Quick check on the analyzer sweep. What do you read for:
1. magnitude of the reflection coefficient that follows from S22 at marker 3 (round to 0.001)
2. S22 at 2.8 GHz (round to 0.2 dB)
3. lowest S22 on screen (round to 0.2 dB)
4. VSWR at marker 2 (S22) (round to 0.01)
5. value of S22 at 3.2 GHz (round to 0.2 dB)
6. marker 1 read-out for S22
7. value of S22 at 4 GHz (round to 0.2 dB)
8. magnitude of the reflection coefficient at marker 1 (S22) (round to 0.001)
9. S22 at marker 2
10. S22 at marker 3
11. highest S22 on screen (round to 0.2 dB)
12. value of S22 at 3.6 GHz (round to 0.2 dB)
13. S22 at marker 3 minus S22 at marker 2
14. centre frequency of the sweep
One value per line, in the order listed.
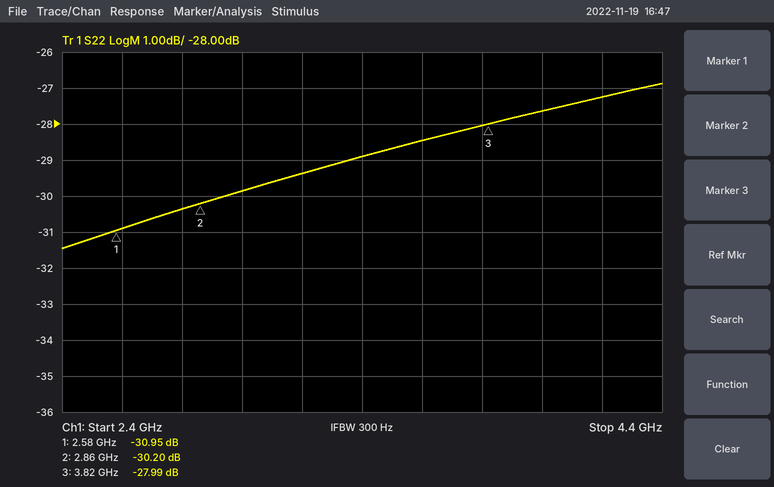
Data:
0.040
-30.4 dB
-31.4 dB
1.06
-29.4 dB
-30.95 dB
-27.6 dB
0.028
-30.20 dB
-27.99 dB
-26.8 dB
-28.4 dB
2.21 dB
3.4 GHz
